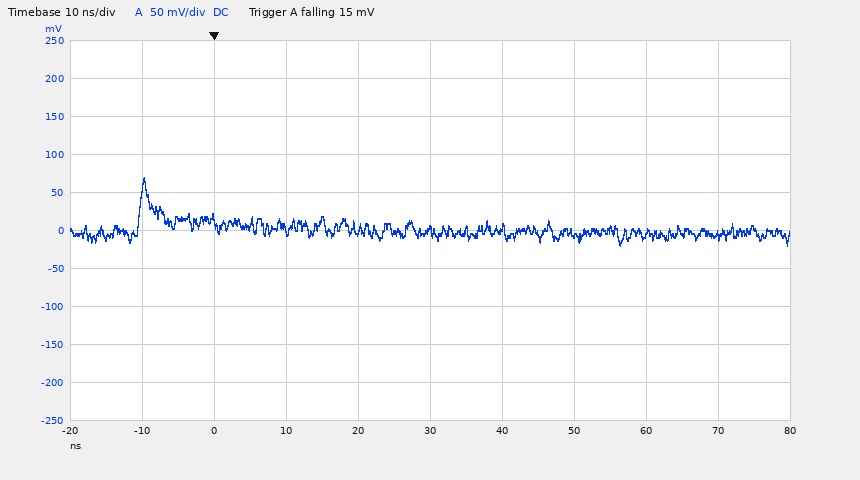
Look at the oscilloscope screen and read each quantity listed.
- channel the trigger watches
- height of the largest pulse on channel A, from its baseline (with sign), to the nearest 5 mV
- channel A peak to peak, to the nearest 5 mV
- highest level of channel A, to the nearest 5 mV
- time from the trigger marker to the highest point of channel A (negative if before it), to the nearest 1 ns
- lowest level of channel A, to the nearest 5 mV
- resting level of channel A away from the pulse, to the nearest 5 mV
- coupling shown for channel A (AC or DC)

channel A
+70 mV
90 mV
70 mV
-10 ns
-20 mV
0 mV
DC
